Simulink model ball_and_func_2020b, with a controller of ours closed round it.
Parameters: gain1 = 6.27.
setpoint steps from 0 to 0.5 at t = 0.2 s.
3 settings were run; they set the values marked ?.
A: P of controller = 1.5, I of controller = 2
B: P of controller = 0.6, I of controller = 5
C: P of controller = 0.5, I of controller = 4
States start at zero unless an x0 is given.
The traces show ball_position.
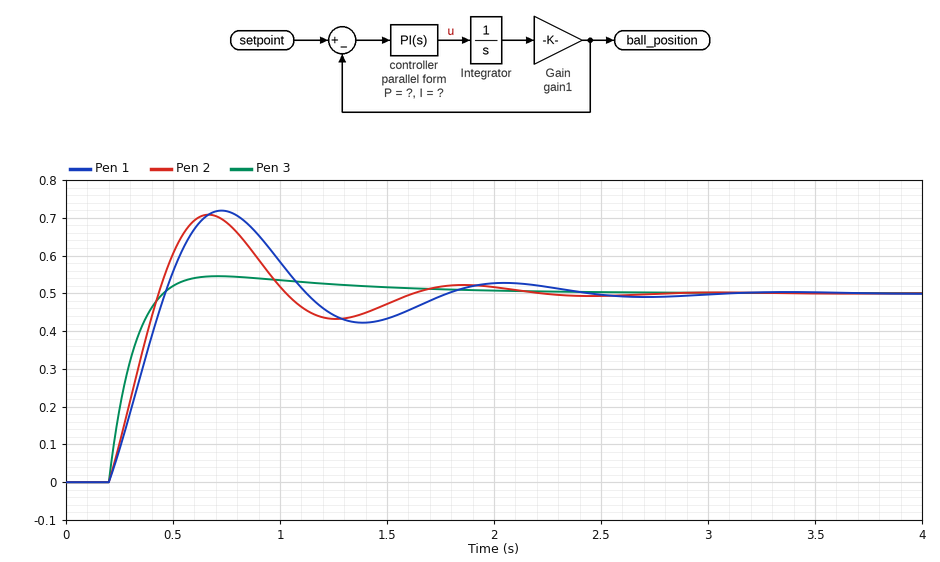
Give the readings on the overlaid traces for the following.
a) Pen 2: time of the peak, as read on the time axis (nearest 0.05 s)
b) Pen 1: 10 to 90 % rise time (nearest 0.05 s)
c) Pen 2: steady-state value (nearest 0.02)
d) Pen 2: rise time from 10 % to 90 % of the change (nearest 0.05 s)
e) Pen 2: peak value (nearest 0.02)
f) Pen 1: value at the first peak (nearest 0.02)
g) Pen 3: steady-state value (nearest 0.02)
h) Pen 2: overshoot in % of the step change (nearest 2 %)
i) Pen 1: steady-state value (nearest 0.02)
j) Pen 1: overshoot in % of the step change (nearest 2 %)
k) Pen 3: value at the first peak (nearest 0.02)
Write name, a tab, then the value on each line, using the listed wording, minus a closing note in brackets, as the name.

Pen 2: time of the peak, as read on the time axis	0.65 s
Pen 1: 10 to 90 % rise time	0.20 s
Pen 2: steady-state value	0.50
Pen 2: rise time from 10 % to 90 % of the change	0.20 s
Pen 2: peak value	0.70
Pen 1: value at the first peak	0.72
Pen 3: steady-state value	0.50
Pen 2: overshoot in % of the step change	42 %
Pen 1: steady-state value	0.50
Pen 1: overshoot in % of the step change	44 %
Pen 3: value at the first peak	0.54
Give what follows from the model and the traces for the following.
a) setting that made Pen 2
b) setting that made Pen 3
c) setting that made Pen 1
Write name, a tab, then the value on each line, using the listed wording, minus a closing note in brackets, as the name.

setting that made Pen 2	B
setting that made Pen 3	A
setting that made Pen 1	C
